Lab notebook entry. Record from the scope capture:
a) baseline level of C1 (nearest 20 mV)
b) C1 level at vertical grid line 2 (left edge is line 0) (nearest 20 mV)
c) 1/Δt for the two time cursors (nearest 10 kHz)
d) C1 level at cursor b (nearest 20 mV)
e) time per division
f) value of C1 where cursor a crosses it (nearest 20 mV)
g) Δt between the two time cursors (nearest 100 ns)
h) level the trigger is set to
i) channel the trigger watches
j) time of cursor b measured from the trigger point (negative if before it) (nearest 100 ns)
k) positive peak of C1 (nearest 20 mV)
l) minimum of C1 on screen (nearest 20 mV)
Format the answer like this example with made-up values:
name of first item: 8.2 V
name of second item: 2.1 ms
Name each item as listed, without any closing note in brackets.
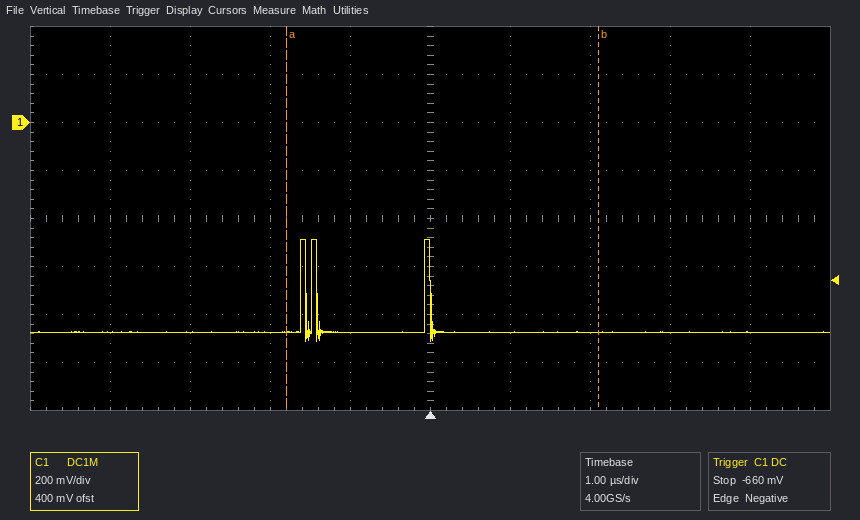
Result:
baseline level of C1: -880 mV
C1 level at vertical grid line 2 (left edge is line 0): -880 mV
1/Δt for the two time cursors: 260 kHz
C1 level at cursor b: -880 mV
time per division: 1 µs
value of C1 where cursor a crosses it: -880 mV
Δt between the two time cursors: 3.9 µs
level the trigger is set to: -660 mV
channel the trigger watches: C1
time of cursor b measured from the trigger point (negative if before it): +2.1 µs
positive peak of C1: -480 mV
minimum of C1 on screen: -920 mV
